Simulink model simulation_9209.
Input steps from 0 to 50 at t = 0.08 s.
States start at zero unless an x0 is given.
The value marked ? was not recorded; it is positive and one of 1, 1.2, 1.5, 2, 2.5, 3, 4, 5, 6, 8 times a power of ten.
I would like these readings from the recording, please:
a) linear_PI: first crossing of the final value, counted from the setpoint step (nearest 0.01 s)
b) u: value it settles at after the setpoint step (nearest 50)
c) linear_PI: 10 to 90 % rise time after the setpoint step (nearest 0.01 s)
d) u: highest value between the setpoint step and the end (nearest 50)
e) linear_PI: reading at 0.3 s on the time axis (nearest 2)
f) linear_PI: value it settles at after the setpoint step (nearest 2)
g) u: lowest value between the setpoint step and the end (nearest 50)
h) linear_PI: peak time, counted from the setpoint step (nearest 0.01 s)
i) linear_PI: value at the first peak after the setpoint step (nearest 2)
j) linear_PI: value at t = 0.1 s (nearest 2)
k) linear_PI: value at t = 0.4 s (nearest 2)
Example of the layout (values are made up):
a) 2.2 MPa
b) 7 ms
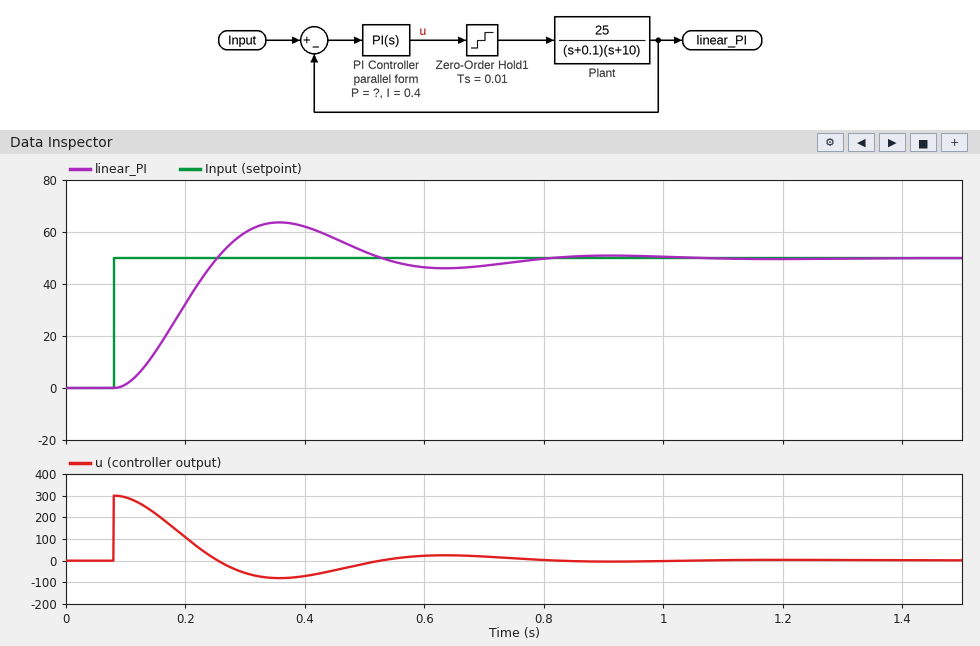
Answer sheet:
a) 0.17 s
b) 0
c) 0.12 s
d) 300
e) 60
f) 50
g) -100
h) 0.28 s
i) 64
j) 2
k) 62
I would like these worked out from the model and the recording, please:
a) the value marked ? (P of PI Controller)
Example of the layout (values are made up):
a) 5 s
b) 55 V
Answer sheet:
a) 6
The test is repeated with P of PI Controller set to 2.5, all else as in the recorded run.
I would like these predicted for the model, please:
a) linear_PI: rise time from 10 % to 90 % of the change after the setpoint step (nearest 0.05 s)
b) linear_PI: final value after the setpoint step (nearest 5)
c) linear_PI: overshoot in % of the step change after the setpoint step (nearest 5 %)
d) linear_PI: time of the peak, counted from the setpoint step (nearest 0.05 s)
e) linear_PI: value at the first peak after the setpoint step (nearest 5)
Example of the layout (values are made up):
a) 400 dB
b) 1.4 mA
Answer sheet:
a) 0.25 s
b) 50
c) 10 %
d) 0.50 s
e) 55
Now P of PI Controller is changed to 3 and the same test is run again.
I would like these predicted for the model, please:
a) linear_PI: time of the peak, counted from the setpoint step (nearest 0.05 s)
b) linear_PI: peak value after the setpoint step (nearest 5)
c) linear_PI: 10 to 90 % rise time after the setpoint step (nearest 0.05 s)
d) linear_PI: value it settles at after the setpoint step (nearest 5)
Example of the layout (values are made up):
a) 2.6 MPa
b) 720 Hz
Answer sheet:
a) 0.45 s
b) 55
c) 0.20 s
d) 50
